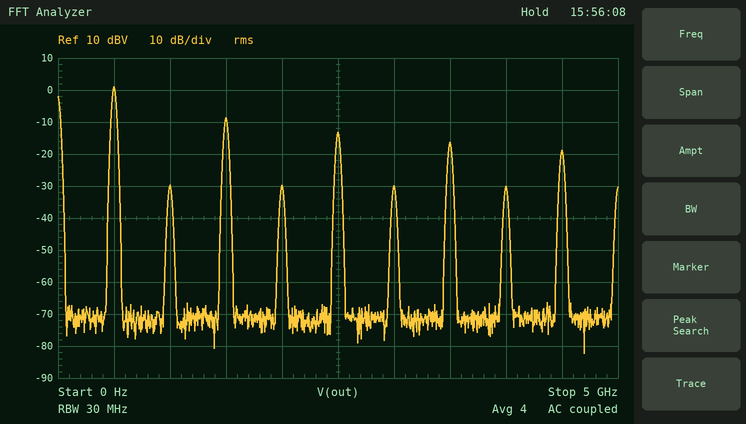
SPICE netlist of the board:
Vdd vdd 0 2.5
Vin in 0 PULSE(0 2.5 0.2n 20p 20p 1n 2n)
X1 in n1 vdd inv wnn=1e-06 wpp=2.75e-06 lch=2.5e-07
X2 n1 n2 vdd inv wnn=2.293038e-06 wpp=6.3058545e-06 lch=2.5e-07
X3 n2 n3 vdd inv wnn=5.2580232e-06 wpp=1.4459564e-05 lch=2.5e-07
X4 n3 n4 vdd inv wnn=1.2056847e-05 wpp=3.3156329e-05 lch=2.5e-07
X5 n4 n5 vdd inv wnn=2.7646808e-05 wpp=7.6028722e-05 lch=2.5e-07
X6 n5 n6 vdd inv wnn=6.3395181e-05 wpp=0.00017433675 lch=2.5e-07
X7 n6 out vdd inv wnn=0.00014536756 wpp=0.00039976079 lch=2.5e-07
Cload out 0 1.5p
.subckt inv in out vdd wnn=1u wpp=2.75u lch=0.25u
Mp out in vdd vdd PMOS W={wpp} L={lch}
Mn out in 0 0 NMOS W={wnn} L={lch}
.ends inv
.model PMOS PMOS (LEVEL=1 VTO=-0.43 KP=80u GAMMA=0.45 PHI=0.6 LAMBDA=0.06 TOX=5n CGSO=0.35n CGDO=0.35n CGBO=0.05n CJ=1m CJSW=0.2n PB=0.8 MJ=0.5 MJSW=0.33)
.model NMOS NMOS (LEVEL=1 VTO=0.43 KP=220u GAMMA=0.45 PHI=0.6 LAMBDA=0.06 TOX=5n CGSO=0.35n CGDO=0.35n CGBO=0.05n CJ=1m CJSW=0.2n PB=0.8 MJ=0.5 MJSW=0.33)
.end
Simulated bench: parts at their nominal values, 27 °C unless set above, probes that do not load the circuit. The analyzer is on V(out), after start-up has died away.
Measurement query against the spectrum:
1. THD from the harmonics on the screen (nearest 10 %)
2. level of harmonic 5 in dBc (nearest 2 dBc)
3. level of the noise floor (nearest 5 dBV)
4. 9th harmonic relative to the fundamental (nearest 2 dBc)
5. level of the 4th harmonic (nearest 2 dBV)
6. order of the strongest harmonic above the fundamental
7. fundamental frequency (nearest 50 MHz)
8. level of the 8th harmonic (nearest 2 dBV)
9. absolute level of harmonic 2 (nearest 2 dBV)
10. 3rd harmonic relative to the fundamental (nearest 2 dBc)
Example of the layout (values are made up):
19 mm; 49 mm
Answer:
40 %; -14 dBc; -70 dBV; -20 dBc; -30 dBV; 3; 500 MHz; -30 dBV; -30 dBV; -10 dBc
